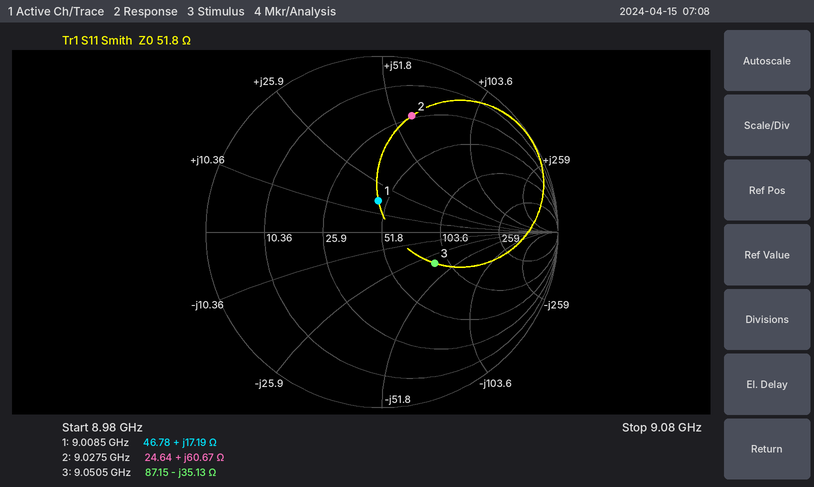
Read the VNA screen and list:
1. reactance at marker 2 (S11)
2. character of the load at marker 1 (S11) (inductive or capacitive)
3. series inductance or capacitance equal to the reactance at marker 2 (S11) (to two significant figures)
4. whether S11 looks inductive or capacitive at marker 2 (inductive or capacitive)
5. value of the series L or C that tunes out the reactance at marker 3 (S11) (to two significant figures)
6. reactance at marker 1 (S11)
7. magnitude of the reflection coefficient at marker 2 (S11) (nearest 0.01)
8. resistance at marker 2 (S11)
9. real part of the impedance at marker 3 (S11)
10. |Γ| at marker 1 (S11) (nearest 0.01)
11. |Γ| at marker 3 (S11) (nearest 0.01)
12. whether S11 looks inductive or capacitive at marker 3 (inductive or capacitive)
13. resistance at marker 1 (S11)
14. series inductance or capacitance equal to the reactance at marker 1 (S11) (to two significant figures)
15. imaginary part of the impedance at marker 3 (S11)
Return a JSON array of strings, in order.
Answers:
["+60.67 Ω", "inductive", "1.1 nH", "inductive", "620 pH", "+17.19 Ω", "0.68", "24.64 Ω", "87.15 Ω", "0.18", "0.35", "capacitive", "46.78 Ω", "300 pH", "-35.13 Ω"]
